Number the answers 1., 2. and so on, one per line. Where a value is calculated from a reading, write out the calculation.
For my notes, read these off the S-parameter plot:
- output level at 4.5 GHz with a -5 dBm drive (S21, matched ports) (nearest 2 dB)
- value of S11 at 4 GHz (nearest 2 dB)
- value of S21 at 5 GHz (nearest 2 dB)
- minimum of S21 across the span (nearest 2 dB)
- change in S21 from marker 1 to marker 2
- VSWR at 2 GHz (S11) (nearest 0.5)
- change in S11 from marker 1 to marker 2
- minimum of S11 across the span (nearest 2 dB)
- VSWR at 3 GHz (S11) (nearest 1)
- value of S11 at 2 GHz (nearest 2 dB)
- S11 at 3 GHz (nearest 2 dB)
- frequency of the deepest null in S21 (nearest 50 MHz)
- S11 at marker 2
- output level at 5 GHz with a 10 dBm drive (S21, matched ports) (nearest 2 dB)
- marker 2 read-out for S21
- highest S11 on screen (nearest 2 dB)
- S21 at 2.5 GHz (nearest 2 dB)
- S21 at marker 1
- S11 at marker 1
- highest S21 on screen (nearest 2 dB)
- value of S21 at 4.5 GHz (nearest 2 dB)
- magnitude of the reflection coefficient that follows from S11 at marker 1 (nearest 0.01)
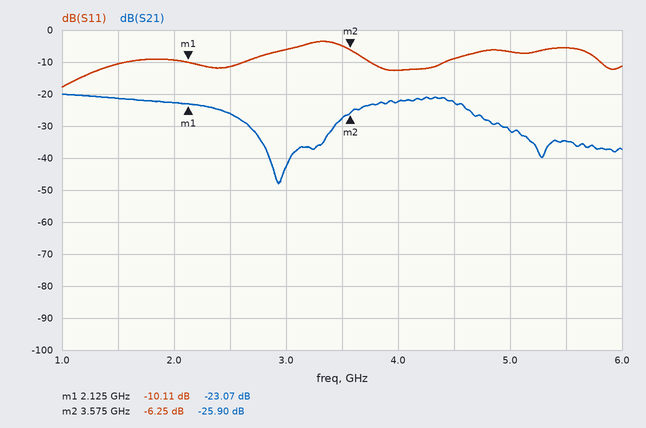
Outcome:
1. -5 dBm + (-22 dB) = -28 dBm
2. -12 dB
3. -32 dB
4. -48 dB
5. -25.9 − (-23.07) = -2.83 dB
6. |Γ| = 10^(-10/20) = 0.3162; VSWR = (1 + 0.3162)/(1 − 0.3162) ≈ 1.92, so 2.0 to the nearest 0.5
7. -6.25 − (-10.11) = 3.86 dB
8. -18 dB
9. |Γ| = 10^(-6/20) = 0.5012; VSWR = (1 + 0.5012)/(1 − 0.5012) ≈ 3
10. -10 dB
11. -6 dB
12. 2.95 GHz
13. -6.25 dB
14. 10 dBm + (-32 dB) = -22 dBm
15. -25.90 dB
16. -4 dB
17. -26 dB
18. -23.07 dB
19. -10.11 dB
20. -20 dB
21. -22 dB
22. 10^(-10.11/20) ≈ 0.31
